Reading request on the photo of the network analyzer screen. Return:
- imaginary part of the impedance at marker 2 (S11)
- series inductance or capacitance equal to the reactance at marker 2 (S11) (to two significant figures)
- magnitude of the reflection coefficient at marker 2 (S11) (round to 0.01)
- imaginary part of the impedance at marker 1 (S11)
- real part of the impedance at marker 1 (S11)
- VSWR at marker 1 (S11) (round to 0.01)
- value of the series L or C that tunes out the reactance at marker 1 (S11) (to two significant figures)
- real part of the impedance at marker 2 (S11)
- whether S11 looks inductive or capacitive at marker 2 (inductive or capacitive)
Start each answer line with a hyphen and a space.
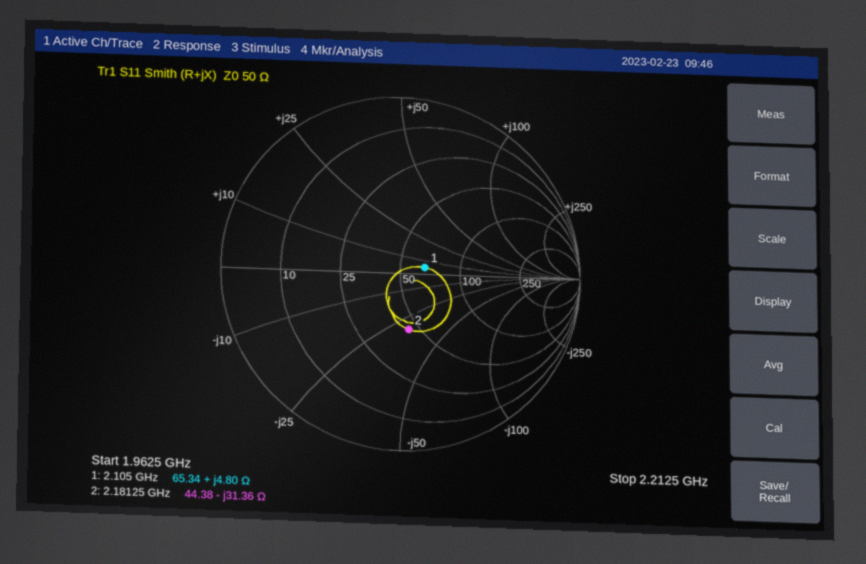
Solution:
- -31.36 Ω
- 2.3 pF
- 0.32
- +4.80 Ω
- 65.34 Ω
- 1.32
- 16 pF
- 44.38 Ω
- capacitive
